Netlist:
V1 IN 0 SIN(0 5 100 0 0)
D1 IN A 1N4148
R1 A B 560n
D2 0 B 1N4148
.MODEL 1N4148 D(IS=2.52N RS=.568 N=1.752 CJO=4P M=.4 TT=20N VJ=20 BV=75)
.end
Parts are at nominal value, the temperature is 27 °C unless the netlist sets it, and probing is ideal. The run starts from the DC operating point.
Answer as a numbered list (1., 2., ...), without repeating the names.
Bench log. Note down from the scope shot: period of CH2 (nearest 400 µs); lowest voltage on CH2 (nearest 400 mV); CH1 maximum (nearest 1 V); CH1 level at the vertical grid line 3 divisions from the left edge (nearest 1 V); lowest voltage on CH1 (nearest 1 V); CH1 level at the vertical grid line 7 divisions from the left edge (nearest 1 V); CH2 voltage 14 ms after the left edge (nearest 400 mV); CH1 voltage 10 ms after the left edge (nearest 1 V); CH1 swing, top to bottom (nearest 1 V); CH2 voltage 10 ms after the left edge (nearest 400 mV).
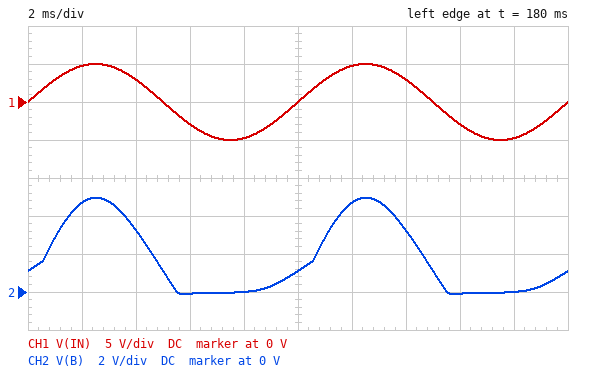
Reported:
1. 10.0 ms
2. 0 V
3. 5 V
4. -3 V
5. -5 V
6. 3 V
7. 3.2 V
8. 0 V
9. 10 V
10. 1.2 V
